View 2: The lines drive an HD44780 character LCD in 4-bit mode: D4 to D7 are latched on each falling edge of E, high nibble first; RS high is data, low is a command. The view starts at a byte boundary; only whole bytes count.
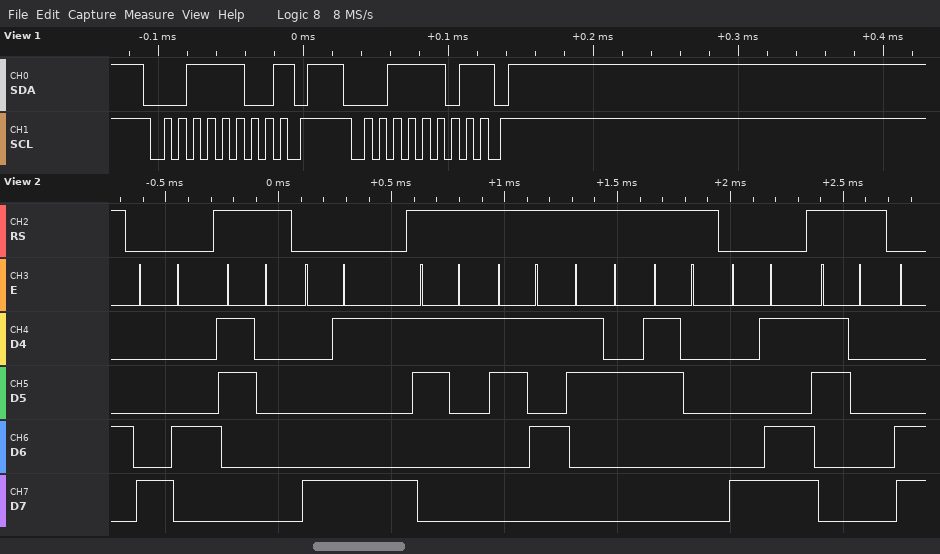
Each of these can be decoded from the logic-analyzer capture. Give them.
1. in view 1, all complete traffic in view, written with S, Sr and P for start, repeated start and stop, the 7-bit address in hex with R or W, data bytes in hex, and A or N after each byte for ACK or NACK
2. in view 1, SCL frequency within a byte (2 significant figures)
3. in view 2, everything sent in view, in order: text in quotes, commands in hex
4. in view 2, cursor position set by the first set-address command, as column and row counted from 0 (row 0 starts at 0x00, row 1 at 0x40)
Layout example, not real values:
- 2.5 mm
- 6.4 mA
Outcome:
- S 1EW N P S 1ER N P
- 100 kHz
- 0x84 "0" 0x89 "1520" 0x8D "0"
- column 4, row 0
